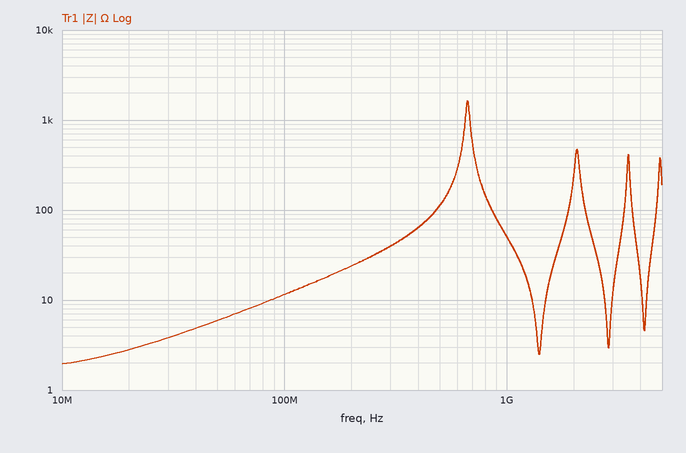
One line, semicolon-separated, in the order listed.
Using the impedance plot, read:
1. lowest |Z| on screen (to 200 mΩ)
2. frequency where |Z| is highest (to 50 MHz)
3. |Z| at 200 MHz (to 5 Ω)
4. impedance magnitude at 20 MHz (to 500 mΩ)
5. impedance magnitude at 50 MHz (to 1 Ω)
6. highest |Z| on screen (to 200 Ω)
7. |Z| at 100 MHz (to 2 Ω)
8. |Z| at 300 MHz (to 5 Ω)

2.0 Ω; 650 MHz; 25 Ω; 3.0 Ω; 6 Ω; 1.6 kΩ; 12 Ω; 40 Ω
